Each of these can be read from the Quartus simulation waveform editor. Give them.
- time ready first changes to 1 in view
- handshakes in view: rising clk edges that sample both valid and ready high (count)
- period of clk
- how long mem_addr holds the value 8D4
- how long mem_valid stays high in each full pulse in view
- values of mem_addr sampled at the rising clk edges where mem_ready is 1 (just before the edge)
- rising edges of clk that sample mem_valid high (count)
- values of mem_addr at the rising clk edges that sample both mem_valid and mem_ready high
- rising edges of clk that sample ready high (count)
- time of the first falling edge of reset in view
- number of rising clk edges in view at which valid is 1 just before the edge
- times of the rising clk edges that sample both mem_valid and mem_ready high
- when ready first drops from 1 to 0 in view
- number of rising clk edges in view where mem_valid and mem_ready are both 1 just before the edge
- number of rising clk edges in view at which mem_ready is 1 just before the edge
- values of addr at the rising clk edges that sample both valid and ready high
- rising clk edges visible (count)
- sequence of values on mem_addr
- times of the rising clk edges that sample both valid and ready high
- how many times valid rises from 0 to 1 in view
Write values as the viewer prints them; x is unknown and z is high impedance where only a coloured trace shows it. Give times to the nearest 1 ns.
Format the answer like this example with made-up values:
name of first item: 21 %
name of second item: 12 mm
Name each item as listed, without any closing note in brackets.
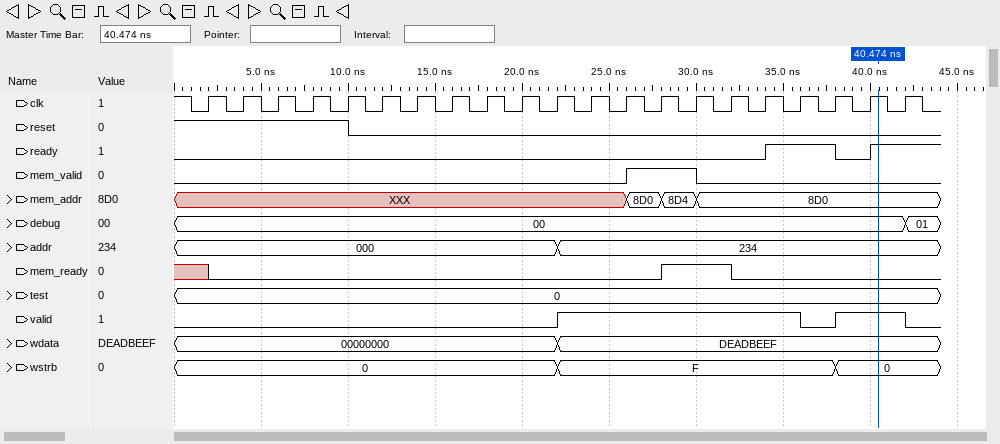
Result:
time ready first changes to 1 in view: 34 ns
handshakes in view: rising clk edges that sample both valid and ready high: 2
period of clk: 2 ns
how long mem_addr holds the value 8D4: 2 ns
how long mem_valid stays high in each full pulse in view: 4 ns
values of mem_addr sampled at the rising clk edges where mem_ready is 1: 8D4, 8D0
rising edges of clk that sample mem_valid high: 2
values of mem_addr at the rising clk edges that sample both mem_valid and mem_ready high: 8D4
rising edges of clk that sample ready high: 3
time of the first falling edge of reset in view: 10 ns
number of rising clk edges in view at which valid is 1 just before the edge: 9
times of the rising clk edges that sample both mem_valid and mem_ready high: 30 ns
when ready first drops from 1 to 0 in view: 38 ns
number of rising clk edges in view where mem_valid and mem_ready are both 1 just before the edge: 1
number of rising clk edges in view at which mem_ready is 1 just before the edge: 2
values of addr at the rising clk edges that sample both valid and ready high: 234, 234
rising clk edges visible: 21
sequence of values on mem_addr: XXX, 8D0, 8D4, 8D0
times of the rising clk edges that sample both valid and ready high: 36 ns, 42 ns
how many times valid rises from 0 to 1 in view: 2
